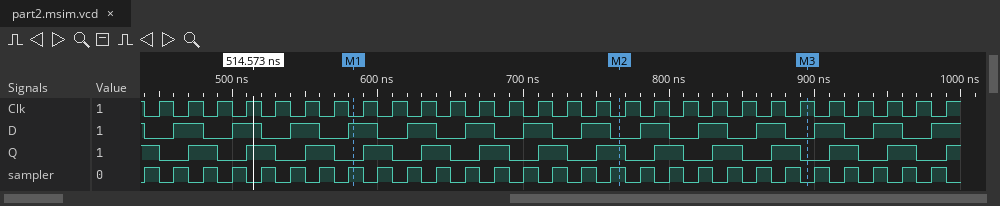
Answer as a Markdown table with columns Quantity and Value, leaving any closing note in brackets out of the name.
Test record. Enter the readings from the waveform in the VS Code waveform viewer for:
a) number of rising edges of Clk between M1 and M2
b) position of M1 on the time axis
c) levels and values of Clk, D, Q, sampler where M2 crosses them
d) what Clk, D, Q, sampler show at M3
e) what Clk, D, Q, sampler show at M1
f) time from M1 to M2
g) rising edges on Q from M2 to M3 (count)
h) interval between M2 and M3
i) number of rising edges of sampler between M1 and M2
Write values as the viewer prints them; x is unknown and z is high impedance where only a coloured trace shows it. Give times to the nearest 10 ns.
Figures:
| Quantity | Value |
|---|---|
| number of rising edges of Clk between M1 and M2 | 9 |
| position of M1 on the time axis | 580 ns |
| levels and values of Clk, D, Q, sampler where M2 crosses them | Clk=0, D=0, Q=1, sampler=1 |
| what Clk, D, Q, sampler show at M3 | Clk=1, D=0, Q=0, sampler=0 |
| what Clk, D, Q, sampler show at M1 | Clk=0, D=1, Q=0, sampler=1 |
| time from M1 to M2 | 180 ns |
| rising edges on Q from M2 to M3 | 3 |
| interval between M2 and M3 | 130 ns |
| number of rising edges of sampler between M1 and M2 | 9 |
